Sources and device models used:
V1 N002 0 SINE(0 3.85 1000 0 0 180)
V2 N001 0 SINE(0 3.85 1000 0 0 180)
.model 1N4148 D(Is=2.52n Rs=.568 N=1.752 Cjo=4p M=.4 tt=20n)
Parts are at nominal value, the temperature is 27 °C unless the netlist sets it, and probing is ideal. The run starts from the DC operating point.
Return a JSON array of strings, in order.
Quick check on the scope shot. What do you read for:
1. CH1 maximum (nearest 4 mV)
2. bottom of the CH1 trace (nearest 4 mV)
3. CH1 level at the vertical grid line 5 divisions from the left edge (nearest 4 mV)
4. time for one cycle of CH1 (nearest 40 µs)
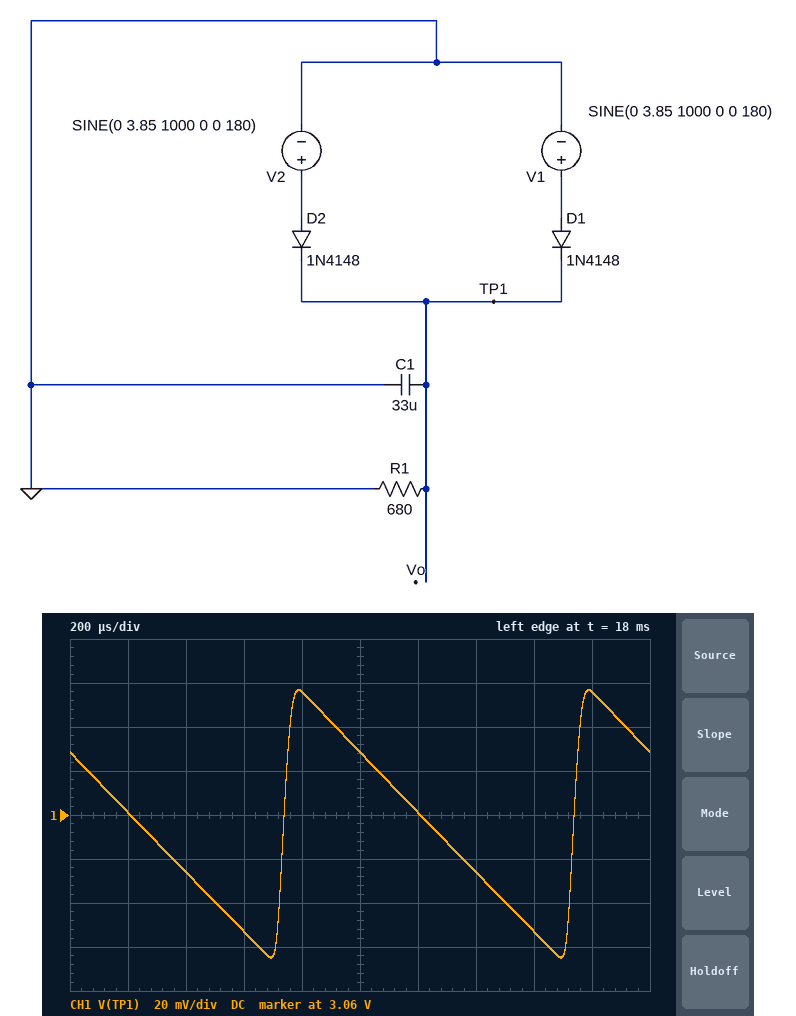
["3.116 V", "2.996 V", "3.088 V", "1.00 ms"]
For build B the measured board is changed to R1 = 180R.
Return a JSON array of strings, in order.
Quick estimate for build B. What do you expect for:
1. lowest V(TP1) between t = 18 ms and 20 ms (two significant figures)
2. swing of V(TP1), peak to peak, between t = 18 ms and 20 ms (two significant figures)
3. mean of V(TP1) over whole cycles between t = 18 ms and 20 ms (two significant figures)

["2.7 V", "420 mV", "2.9 V"]
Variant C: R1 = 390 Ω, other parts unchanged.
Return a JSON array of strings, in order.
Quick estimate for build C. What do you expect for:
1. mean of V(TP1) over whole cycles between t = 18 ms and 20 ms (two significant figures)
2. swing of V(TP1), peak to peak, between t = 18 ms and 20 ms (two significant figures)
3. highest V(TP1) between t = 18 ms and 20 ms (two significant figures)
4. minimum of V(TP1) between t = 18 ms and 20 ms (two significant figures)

["3.0 V", "210 mV", "3.1 V", "2.9 V"]
